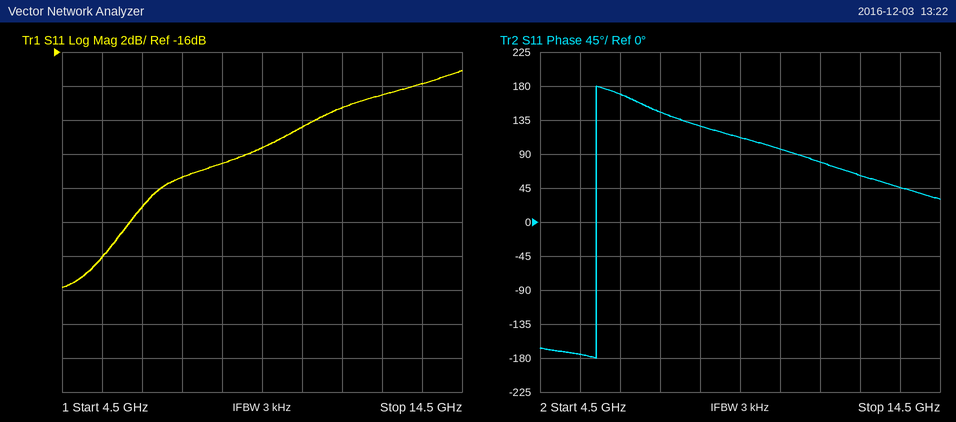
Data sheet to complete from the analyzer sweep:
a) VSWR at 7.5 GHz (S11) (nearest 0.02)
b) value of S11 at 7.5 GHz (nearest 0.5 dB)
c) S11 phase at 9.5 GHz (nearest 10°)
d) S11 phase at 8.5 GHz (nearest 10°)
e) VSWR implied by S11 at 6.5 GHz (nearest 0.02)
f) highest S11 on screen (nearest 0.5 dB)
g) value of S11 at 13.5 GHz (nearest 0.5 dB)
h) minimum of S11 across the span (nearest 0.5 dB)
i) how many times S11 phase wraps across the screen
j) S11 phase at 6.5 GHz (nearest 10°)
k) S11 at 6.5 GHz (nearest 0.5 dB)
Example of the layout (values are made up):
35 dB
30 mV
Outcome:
1.14
-23.5 dB
110°
130°
1.12
-17.0 dB
-18.0 dB
-30.0 dB
1
170°
-25.0 dB
